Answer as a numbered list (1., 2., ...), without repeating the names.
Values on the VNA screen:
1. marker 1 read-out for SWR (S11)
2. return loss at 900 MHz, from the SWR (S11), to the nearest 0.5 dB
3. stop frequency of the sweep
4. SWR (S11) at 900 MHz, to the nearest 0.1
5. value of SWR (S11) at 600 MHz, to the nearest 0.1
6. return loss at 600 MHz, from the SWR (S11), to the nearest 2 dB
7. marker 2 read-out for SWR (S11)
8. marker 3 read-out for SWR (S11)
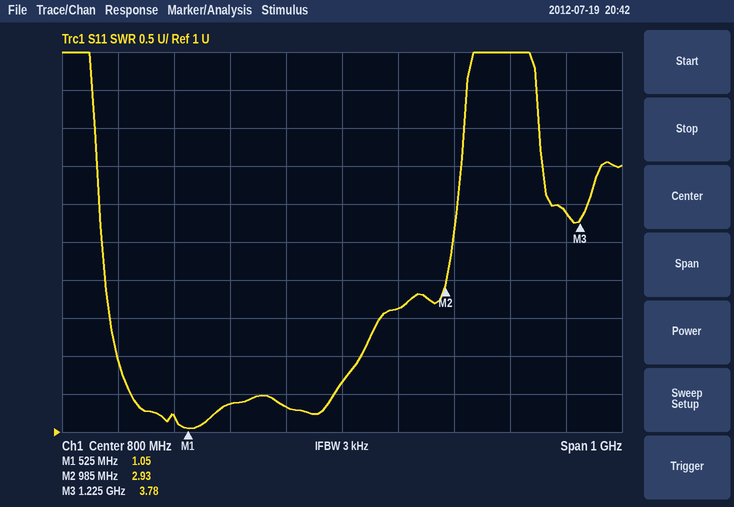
1. 1.05
2. 7.0 dB
3. 1.3 GHz
4. 2.6
5. 1.4
6. 16 dB
7. 2.93
8. 3.78
